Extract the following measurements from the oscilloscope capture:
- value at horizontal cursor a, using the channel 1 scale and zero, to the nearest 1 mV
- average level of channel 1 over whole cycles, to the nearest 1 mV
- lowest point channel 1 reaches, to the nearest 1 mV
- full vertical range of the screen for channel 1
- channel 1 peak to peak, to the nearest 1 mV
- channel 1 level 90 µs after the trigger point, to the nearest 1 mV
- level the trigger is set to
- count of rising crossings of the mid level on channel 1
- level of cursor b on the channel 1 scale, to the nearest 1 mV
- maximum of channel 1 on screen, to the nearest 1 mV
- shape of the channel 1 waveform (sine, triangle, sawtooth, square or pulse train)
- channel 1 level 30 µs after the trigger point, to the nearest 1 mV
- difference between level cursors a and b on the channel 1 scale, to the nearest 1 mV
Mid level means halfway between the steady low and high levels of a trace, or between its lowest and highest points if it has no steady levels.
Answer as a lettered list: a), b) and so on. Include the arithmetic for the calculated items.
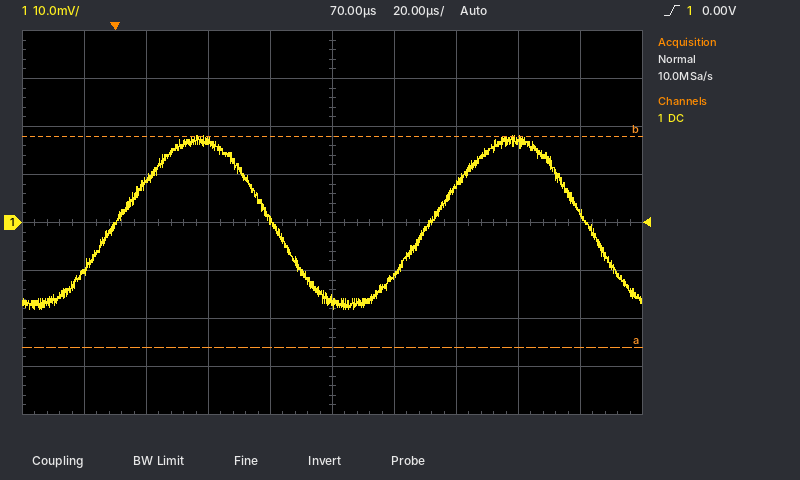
a) -26 mV
b) (18 mV + (-18 mV)) / 2 ≈ 0 mV
c) -18 mV
d) 80 mV
e) 18 mV − (-18 mV) = 36 mV
f) -11 mV
g) 0.00 V
h) 2
i) 18 mV
j) 18 mV
k) sine
l) 17 mV
m) 44 mV
